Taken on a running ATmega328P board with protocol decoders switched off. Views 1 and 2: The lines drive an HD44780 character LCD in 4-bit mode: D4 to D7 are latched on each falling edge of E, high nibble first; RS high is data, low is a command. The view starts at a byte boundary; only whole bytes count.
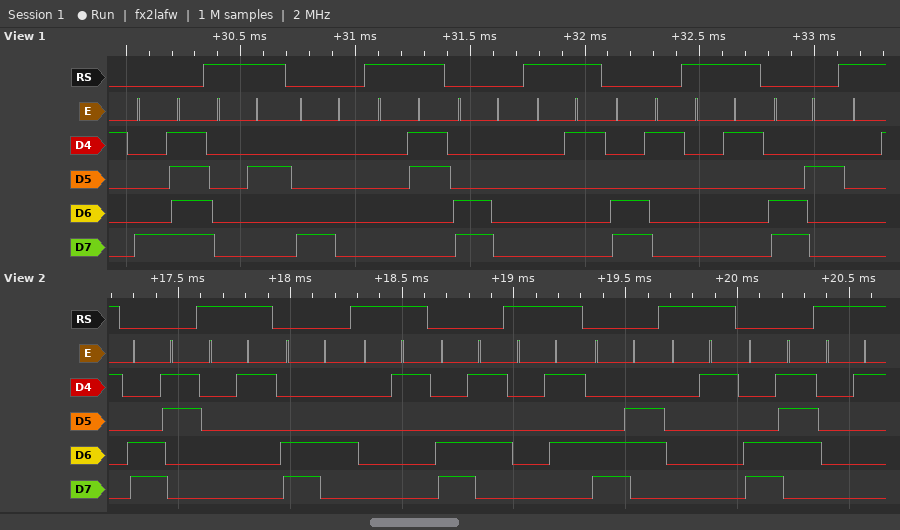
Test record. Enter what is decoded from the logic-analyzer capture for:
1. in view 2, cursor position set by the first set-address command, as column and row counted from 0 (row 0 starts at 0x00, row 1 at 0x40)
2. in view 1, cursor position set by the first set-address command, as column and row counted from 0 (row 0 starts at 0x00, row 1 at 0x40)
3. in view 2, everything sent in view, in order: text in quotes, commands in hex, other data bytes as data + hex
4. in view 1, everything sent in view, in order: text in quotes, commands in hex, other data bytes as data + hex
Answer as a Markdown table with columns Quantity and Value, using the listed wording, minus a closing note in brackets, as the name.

| Quantity | Value |
|---|---|
| in view 2, cursor position set by the first set-address command, as column and row counted from 0 | column 3, row 1 |
| in view 1, cursor position set by the first set-address command, as column and row counted from 0 | column 15, row 0 |
| in view 2, everything sent in view, in order: text in quotes, commands in hex, other data bytes as data + hex | 0xC3 data 01 0xC4 data 01 0xC5 data 05 0xC6 data 01 0xC7 data 01 |
| in view 1, everything sent in view, in order: text in quotes, commands in hex, other data bytes as data + hex | 0x8F data 02 0x80 data 03 0xC0 data 01 0xC1 data 01 0xC2 |
